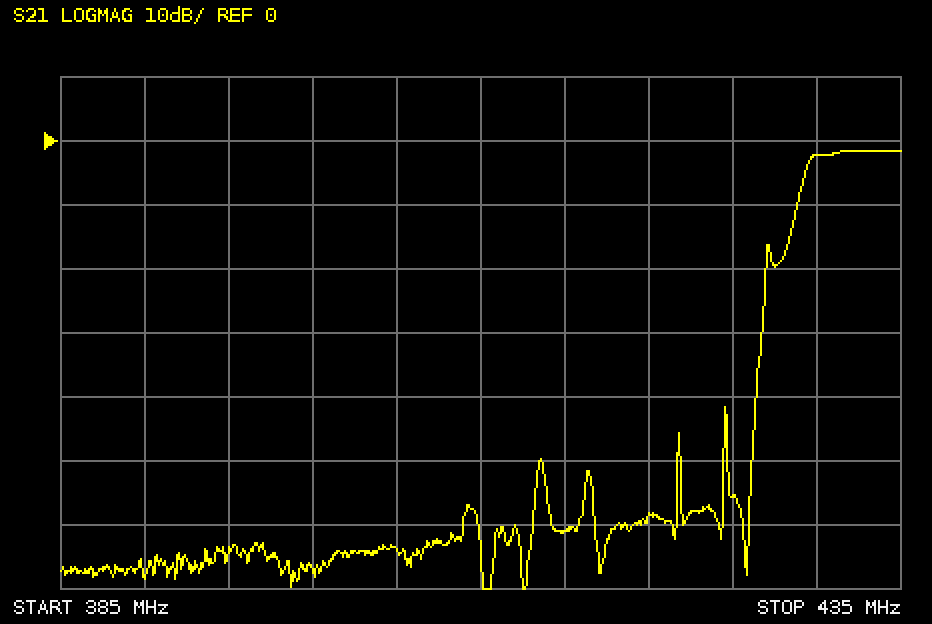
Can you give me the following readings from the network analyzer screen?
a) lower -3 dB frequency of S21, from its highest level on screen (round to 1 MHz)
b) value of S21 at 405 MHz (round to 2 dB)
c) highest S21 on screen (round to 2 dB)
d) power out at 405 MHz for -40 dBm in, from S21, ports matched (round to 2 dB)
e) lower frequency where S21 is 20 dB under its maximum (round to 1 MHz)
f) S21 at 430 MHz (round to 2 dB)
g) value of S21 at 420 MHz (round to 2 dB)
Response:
429 MHz
-64 dB
-2 dB
-104 dBm
427 MHz
-2 dB
-58 dB
